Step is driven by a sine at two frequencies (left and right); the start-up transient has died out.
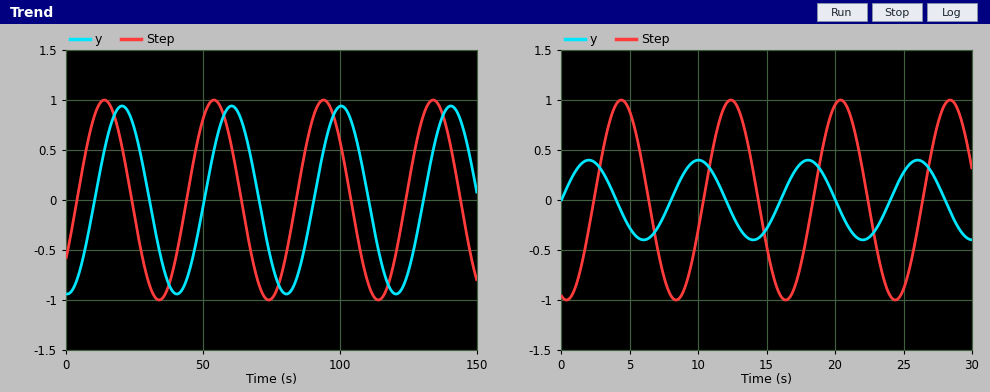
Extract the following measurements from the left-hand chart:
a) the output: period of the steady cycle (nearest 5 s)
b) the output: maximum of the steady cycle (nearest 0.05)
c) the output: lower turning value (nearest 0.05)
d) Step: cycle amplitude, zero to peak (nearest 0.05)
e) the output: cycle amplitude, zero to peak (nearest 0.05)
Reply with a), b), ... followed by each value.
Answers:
a) 40 s
b) 0.95
c) -0.95
d) 1.00
e) 0.95
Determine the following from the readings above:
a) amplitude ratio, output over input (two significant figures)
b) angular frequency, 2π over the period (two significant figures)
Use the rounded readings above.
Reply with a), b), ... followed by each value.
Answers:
a) 0.95
b) 0.16 rad/s
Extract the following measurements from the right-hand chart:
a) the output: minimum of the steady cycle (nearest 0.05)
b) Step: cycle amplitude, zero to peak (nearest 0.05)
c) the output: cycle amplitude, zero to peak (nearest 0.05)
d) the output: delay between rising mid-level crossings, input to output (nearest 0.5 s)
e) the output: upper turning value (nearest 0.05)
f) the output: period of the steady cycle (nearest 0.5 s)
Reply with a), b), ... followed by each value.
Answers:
a) -0.40
b) 1.00
c) 0.40
d) 5.5 s
e) 0.40
f) 8.0 s
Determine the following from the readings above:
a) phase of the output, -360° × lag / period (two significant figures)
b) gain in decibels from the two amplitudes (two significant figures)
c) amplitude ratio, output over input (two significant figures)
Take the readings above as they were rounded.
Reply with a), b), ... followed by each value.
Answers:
a) -250°
b) -8.0 dB
c) 0.40
